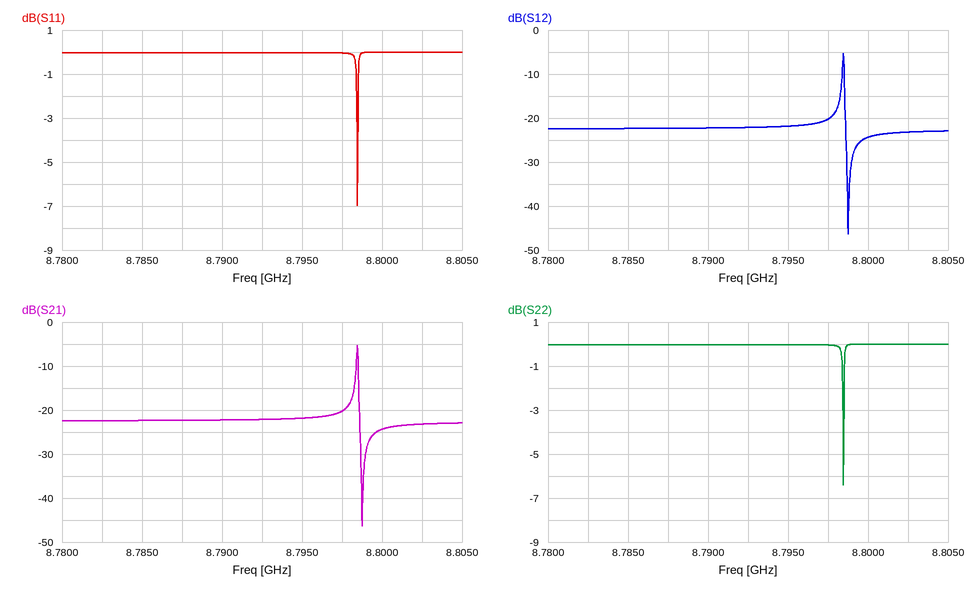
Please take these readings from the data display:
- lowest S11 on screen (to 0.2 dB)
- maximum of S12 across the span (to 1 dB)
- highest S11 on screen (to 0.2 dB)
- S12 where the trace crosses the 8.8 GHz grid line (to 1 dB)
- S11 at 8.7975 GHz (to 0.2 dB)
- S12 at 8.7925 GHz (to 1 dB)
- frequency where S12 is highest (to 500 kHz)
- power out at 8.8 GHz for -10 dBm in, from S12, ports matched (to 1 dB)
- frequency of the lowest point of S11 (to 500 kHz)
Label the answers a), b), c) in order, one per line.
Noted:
a) -7.0 dB
b) -5 dB
c) 0.0 dB
d) -24 dB
e) 0.0 dB
f) -22 dB
g) 8.7985 GHz
h) -34 dBm
i) 8.7985 GHz
